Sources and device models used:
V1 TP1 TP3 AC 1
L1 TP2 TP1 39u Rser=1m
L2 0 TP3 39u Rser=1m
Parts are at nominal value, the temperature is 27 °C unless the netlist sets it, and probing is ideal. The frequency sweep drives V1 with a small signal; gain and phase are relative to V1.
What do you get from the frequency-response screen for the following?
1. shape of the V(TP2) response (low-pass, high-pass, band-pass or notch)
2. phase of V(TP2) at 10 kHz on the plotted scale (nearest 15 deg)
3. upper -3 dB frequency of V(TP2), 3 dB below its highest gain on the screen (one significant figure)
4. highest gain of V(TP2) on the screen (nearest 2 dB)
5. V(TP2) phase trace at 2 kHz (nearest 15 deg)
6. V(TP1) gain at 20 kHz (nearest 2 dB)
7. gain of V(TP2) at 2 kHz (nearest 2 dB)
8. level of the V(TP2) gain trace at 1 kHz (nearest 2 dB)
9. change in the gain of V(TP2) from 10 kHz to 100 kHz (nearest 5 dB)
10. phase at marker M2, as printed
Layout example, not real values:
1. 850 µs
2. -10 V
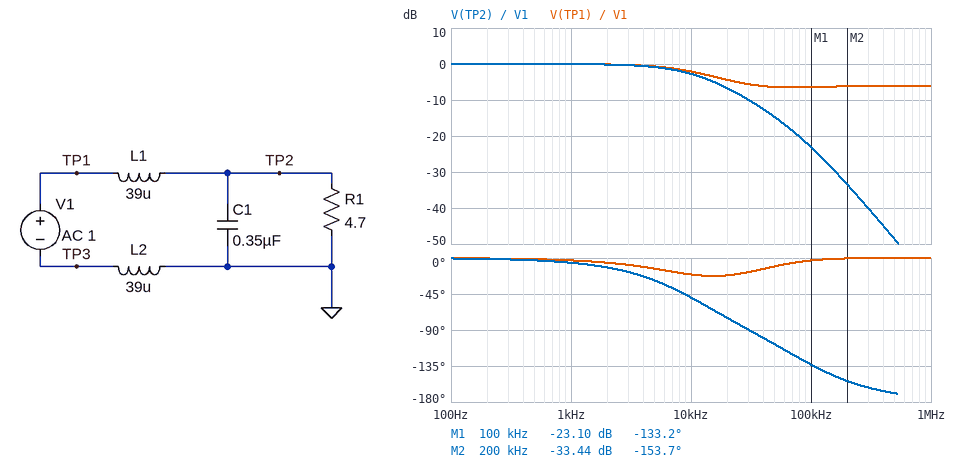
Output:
1. low-pass
2. -45 deg
3. 10 kHz
4. 0 dB
5. -15 deg
6. -4 dB
7. 0 dB
8. 0 dB
9. -20 dB
10. -153.7 deg
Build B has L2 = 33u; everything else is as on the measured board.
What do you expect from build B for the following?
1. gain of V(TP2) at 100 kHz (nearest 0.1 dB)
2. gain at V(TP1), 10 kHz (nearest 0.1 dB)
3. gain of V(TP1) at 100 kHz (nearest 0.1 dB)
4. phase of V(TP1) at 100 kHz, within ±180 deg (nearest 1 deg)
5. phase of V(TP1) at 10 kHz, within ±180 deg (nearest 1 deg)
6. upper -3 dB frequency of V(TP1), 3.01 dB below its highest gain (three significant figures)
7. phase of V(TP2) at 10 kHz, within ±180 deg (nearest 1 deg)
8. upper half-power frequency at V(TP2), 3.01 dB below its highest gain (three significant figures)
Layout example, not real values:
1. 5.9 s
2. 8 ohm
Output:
1. -22.4 dB
2. -1.7 dB
3. -5.7 dB
4. -3 deg
5. -18 deg
6. 15.6 kHz
7. -47 deg
8. 11.6 kHz
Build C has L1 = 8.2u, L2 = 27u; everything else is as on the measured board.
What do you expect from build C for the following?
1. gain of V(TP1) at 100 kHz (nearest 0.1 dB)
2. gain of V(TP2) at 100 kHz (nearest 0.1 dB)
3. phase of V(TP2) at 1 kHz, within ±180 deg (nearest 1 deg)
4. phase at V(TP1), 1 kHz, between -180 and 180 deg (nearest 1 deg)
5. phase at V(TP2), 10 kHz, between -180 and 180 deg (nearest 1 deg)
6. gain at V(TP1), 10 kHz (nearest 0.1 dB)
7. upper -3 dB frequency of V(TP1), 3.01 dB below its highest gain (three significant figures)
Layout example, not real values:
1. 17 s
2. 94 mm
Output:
1. -14.8 dB
2. -15.7 dB
3. -3 deg
4. -2 deg
5. -26 deg
6. -0.6 dB
7. 25.1 kHz
